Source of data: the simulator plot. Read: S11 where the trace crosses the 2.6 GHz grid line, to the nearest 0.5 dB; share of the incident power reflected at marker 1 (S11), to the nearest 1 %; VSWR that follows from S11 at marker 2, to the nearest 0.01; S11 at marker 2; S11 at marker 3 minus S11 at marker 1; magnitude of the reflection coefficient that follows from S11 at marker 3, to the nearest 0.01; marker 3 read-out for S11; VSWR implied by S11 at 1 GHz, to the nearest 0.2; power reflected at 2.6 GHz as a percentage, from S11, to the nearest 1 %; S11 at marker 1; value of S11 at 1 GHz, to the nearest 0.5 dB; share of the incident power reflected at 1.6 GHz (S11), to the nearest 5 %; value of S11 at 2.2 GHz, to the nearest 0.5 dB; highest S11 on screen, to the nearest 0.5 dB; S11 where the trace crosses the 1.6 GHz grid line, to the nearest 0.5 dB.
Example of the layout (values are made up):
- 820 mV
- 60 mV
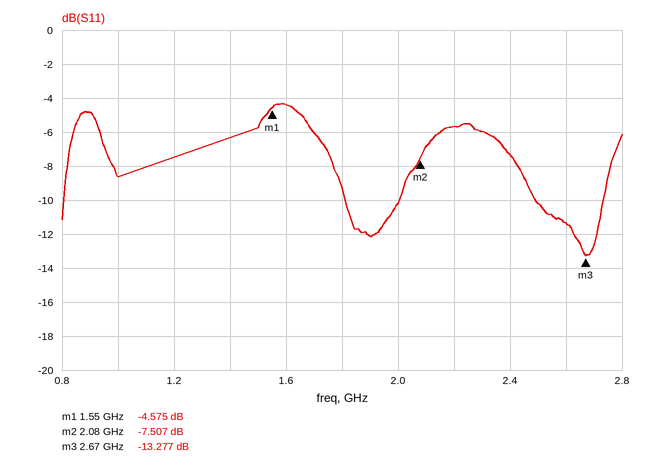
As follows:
- -11.5 dB
- 35 %
- 2.46
- -7.507 dB
- -8.702 dB
- 0.22
- -13.277 dB
- 2.2
- 7 %
- -4.575 dB
- -8.5 dB
- 35 %
- -5.5 dB
- -4.5 dB
- -4.5 dB
